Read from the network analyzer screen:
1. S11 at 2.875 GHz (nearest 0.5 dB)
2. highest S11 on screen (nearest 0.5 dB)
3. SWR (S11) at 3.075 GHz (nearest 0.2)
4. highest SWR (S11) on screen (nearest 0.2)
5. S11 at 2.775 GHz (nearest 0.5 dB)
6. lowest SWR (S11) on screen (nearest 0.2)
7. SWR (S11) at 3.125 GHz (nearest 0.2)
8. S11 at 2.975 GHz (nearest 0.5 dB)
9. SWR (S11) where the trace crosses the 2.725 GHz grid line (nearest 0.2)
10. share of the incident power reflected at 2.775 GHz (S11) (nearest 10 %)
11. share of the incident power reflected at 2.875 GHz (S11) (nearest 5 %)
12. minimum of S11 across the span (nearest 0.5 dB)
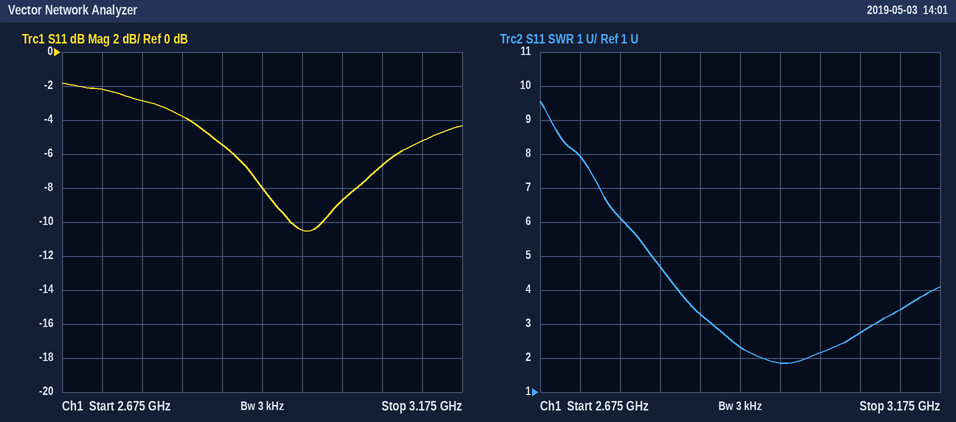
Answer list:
-5.5 dB
-2.0 dB
2.8
9.6
-3.0 dB
1.8
3.4
-10.5 dB
8.0
50 %
30 %
-10.5 dB
